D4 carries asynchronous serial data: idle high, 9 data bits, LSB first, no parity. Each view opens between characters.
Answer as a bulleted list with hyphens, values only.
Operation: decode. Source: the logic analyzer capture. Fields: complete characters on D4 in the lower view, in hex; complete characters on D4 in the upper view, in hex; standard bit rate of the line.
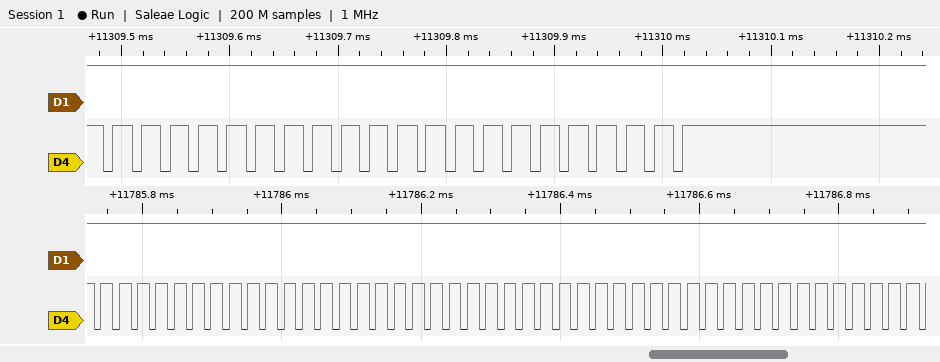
- DB, DB, DB, DB, DB, DB, DB, DB, DB, DB, DB
- DB, DB, DB, DB, DB, 1FF
- 115200 baud
